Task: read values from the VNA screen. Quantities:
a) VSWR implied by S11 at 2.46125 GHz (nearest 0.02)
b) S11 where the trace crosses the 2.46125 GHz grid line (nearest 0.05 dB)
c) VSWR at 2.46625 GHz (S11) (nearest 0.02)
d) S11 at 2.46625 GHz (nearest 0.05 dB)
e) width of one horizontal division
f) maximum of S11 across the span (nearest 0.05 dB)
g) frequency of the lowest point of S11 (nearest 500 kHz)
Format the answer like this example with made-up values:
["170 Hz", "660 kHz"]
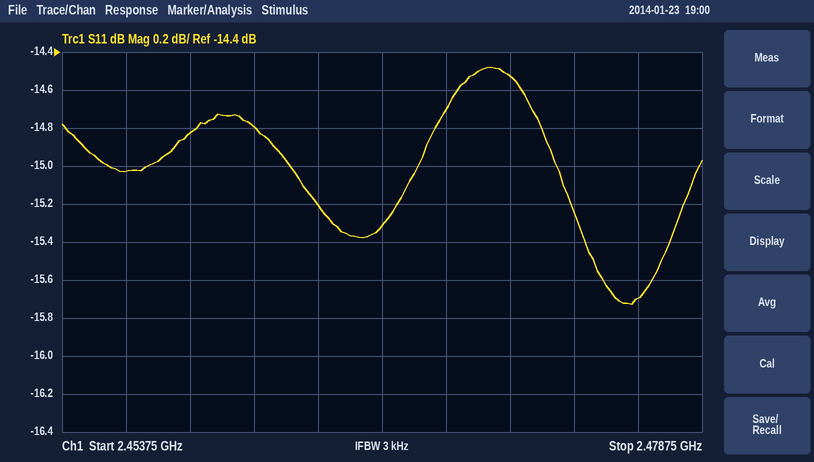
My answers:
["1.44", "-14.80 dB", "1.42", "-15.30 dB", "2.5 MHz", "-14.50 dB", "2.4760 GHz"]
